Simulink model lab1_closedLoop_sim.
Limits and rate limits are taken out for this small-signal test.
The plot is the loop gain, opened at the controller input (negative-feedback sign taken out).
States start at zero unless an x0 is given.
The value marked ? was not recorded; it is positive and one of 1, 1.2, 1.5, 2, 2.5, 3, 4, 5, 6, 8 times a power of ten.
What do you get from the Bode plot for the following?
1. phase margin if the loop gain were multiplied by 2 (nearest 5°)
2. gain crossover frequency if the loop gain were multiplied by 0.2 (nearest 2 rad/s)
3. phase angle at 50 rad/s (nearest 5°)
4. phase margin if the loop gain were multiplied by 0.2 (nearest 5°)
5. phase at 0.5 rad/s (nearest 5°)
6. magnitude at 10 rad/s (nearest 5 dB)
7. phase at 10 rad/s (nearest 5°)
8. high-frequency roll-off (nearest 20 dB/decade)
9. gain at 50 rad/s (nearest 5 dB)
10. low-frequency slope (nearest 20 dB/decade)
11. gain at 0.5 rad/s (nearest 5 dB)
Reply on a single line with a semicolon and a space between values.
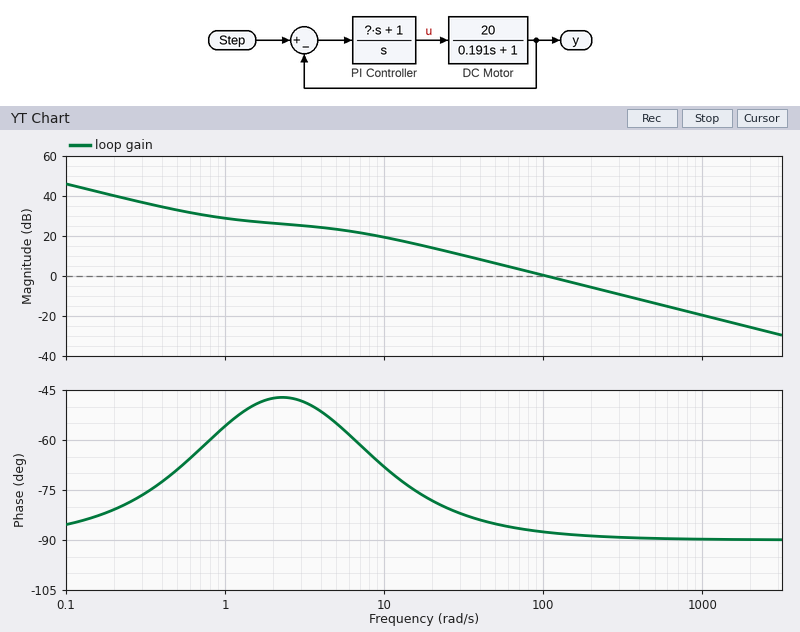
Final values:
90°; 20 rad/s; -85°; 100°; -70°; 20 dB; -70°; -20 dB/decade; 5 dB; -20 dB/decade; 35 dB
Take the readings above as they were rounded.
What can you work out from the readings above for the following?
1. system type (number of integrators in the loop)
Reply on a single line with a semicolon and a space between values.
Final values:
1
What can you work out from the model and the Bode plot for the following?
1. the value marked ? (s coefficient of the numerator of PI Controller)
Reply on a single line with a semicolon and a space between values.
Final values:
1
